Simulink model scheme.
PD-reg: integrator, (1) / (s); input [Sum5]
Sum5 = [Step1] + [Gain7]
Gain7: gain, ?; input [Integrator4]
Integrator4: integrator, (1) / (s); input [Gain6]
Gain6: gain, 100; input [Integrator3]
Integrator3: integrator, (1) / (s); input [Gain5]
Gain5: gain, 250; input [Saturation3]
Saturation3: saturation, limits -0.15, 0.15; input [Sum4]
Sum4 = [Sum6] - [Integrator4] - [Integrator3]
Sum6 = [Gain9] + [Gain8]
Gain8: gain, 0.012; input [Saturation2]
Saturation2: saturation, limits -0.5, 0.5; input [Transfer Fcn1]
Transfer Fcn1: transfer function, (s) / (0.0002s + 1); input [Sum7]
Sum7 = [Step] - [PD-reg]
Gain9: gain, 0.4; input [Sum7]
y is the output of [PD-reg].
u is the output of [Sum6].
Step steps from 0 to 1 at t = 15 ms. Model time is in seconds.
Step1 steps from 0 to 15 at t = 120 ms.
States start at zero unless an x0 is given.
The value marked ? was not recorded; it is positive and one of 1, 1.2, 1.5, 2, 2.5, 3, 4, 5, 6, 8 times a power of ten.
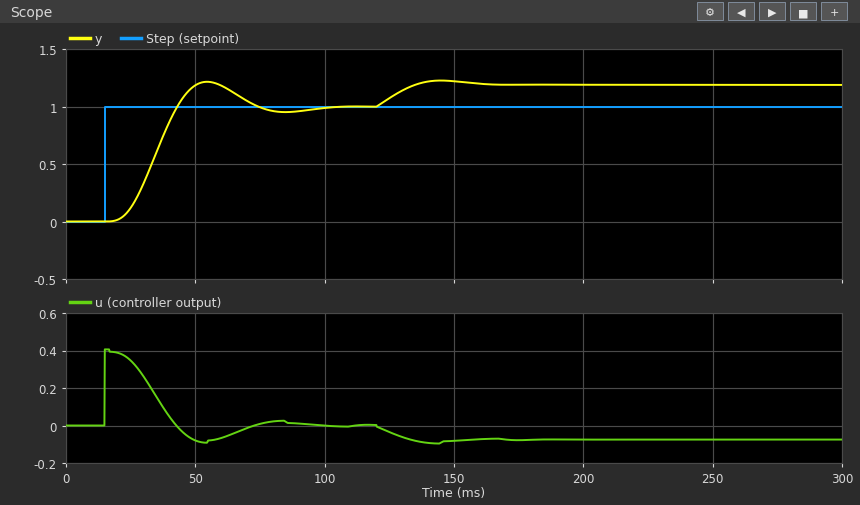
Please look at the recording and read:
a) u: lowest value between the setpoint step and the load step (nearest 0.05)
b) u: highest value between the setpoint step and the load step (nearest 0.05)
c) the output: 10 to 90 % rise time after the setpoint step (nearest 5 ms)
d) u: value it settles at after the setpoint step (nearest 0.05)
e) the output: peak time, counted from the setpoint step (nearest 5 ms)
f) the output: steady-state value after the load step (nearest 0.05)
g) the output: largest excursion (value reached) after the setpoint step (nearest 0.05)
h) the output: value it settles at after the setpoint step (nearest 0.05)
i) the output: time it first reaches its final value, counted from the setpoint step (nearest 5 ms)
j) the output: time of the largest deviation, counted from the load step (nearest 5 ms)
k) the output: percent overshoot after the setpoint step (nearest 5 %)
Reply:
-0.10
0.40
15 ms
0.00
40 ms
1.20
1.20
1.00
30 ms
25 ms
20 %
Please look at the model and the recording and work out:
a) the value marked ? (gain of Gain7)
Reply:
200
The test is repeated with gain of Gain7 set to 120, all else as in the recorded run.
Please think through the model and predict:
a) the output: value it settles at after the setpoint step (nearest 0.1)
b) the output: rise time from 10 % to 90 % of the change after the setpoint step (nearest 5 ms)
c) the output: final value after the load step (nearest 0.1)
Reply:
1.0
25 ms
1.3
